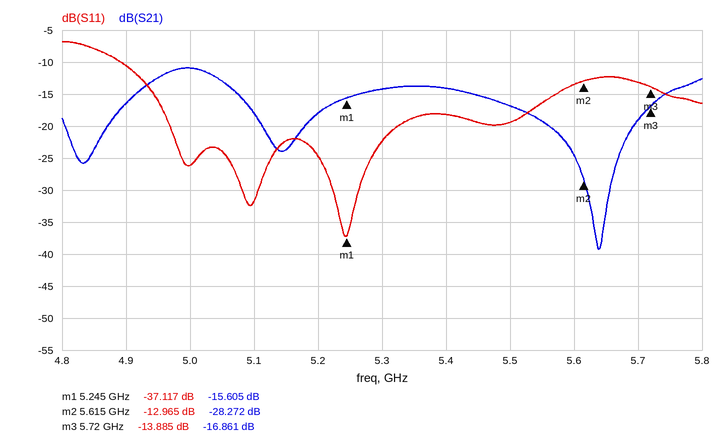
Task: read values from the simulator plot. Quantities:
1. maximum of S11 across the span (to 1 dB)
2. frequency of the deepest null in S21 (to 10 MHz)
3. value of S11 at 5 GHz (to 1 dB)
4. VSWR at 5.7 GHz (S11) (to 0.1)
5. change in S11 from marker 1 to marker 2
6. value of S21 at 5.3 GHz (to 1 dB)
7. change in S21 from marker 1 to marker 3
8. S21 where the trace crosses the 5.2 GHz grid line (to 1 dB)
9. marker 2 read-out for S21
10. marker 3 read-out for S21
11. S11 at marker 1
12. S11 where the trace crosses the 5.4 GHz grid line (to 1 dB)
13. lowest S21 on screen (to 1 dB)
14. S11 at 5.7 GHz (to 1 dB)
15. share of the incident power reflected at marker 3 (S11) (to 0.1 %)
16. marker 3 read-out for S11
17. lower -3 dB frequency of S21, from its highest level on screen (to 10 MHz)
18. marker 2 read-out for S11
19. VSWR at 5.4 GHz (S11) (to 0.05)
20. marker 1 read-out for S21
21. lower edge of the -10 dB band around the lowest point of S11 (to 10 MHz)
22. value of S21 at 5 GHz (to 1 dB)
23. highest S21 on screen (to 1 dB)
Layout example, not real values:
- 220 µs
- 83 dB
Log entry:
- -7 dB
- 5.64 GHz
- -26 dB
- 1.6
- 24.152 dB
- -14 dB
- -1.256 dB
- -18 dB
- -28.272 dB
- -16.861 dB
- -37.117 dB
- -18 dB
- -39 dB
- -13 dB
- 4.1 %
- -13.885 dB
- 4.93 GHz
- -12.965 dB
- 1.30
- -15.605 dB
- 4.89 GHz
- -11 dB
- -11 dB
